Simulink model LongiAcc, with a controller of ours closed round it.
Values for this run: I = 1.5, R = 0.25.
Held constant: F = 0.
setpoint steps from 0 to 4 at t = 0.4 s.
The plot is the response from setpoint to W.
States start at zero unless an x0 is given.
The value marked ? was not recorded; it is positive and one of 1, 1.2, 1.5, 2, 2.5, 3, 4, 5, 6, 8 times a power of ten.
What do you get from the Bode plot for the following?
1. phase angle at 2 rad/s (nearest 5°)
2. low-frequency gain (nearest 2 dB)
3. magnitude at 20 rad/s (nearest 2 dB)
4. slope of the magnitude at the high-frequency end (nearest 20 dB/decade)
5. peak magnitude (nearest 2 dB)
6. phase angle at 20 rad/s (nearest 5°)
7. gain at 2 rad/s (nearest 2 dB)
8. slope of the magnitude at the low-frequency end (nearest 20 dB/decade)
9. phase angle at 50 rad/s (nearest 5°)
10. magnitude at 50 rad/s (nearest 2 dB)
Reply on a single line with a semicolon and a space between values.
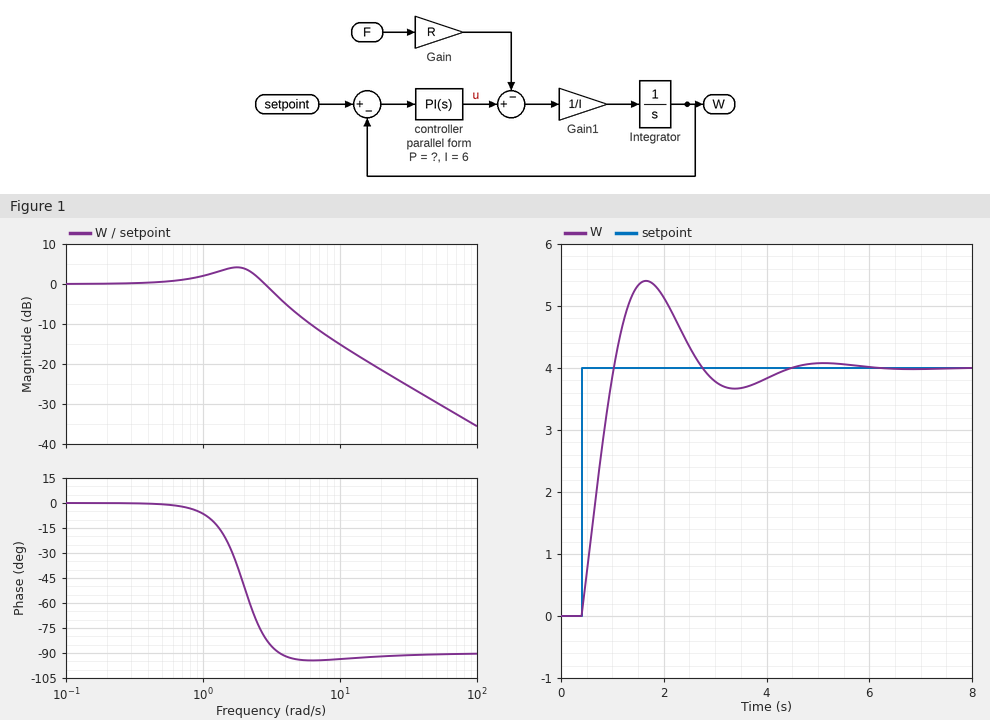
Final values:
-50°; 0 dB; -22 dB; -20 dB/decade; 4 dB; -90°; 4 dB; 0 dB/decade; -90°; -30 dB
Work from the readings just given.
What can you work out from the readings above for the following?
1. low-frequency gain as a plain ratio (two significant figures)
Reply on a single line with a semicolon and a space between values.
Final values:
1.0
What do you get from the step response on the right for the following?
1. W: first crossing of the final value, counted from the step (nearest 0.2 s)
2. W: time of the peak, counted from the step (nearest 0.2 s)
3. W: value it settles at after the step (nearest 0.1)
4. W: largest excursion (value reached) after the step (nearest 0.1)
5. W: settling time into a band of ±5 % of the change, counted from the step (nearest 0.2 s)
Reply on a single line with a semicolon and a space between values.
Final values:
0.6 s; 1.2 s; 4.0; 5.4; 3.6 s
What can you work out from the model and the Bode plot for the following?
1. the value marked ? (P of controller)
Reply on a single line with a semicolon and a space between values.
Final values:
2.5
